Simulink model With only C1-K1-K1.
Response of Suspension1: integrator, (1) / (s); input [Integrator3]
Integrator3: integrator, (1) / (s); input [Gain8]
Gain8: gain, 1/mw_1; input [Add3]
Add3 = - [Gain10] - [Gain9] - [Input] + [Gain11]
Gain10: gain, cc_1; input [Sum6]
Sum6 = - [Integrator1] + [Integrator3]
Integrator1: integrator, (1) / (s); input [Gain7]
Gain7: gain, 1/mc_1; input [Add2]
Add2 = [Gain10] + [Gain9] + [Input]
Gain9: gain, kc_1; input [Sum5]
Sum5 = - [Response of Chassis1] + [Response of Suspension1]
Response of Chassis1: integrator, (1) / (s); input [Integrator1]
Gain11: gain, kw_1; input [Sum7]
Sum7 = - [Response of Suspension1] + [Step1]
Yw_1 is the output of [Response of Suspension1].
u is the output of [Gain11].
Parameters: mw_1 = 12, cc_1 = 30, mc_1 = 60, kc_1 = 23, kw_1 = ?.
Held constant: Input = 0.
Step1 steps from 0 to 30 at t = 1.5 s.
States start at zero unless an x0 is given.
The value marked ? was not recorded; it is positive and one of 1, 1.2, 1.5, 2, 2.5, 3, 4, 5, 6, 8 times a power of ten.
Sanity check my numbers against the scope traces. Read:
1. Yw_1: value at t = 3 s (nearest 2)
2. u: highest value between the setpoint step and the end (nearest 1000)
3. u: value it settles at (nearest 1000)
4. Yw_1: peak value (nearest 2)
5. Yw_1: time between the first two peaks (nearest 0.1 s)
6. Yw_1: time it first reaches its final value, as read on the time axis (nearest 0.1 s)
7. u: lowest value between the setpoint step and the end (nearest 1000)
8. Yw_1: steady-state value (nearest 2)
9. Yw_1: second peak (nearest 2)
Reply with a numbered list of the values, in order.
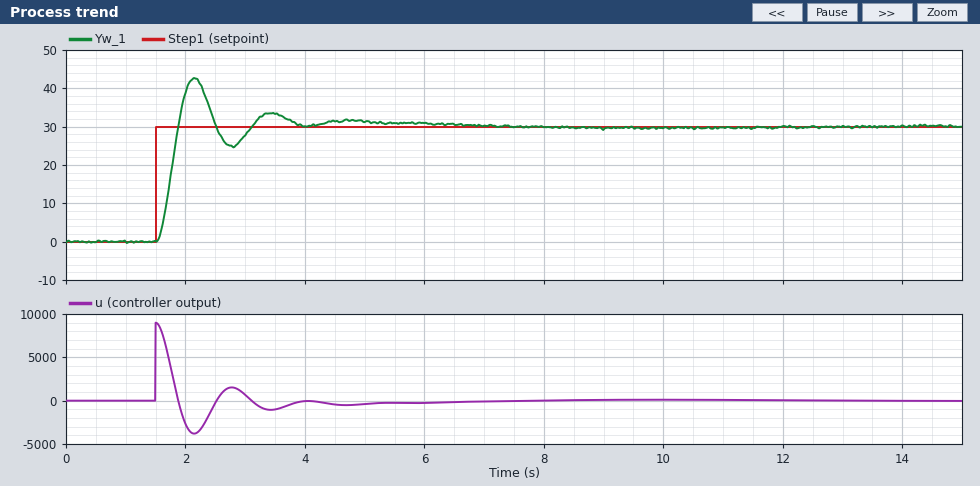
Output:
1. 28
2. 9000
3. 0
4. 42
5. 1.3 s
6. 1.9 s
7. -4000
8. 30
9. 34
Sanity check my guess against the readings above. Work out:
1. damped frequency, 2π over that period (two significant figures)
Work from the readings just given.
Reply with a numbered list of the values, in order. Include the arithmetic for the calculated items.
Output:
1. 2π / 1.3 = 4.8 rad/s
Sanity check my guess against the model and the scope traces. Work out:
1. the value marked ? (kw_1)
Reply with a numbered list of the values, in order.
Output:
1. 300
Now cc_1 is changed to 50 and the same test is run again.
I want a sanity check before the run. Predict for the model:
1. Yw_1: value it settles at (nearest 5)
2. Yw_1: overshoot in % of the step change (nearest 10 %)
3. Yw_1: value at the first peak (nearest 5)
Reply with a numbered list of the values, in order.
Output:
1. 30
2. 30 %
3. 40
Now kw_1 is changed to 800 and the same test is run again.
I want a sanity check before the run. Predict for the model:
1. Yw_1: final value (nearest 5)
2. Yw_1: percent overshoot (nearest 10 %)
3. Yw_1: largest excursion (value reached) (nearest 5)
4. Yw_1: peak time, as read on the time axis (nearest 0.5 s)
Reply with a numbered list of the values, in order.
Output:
1. 30
2. 60 %
3. 50
4. 2.0 s
